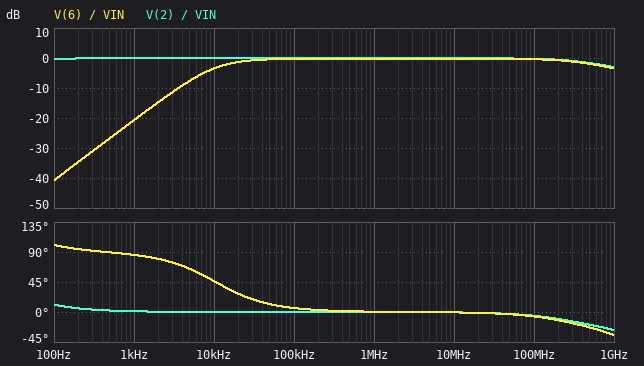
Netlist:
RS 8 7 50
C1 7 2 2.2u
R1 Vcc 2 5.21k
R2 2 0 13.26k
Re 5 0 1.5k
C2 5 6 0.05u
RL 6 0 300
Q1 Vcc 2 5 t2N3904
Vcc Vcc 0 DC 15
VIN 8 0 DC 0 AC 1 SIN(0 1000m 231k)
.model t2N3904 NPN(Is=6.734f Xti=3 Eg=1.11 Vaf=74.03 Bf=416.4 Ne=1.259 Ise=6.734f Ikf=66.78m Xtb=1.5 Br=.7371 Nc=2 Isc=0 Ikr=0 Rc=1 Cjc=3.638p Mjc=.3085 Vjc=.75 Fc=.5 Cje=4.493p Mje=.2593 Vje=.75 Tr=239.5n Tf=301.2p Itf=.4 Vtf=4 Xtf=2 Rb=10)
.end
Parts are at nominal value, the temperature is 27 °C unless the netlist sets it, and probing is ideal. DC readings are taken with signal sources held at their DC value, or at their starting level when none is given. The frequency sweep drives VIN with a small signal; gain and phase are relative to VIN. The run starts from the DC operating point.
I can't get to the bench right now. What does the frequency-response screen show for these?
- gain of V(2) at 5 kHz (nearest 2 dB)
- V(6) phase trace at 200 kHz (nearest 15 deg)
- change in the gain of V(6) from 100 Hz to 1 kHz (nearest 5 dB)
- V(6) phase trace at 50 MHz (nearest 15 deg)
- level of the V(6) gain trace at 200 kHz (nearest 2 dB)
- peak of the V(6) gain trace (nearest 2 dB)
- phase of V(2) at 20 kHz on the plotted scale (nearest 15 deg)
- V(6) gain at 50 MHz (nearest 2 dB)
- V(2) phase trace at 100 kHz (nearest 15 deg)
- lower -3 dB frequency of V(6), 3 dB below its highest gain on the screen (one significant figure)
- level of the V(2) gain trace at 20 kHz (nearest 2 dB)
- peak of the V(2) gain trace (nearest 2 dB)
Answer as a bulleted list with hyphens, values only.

- 0 dB
- 0 deg
- 20 dB
- 0 deg
- 0 dB
- 0 dB
- 0 deg
- 0 dB
- 0 deg
- 10 kHz
- 0 dB
- 0 dB
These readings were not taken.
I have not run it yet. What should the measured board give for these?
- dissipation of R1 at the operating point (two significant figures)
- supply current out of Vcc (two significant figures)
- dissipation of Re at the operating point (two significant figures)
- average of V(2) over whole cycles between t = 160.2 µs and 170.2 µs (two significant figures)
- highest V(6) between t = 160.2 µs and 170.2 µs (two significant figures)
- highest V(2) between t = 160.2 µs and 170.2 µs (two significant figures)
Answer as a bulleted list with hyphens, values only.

- 3.7 mW
- 7.4 mA
- 65 mW
- 11 V
- 970 mV
- 12 V
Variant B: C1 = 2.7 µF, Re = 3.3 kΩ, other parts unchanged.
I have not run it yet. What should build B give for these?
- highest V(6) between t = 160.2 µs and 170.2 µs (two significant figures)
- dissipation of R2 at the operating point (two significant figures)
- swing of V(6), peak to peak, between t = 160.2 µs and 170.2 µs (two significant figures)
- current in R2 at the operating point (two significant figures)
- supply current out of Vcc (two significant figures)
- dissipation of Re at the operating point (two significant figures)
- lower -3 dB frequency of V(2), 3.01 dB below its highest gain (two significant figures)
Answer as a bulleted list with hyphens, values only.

- 940 mV
- 8.6 mW
- 1.8 V
- 810 µA
- 3.8 mA
- 30 mW
- 16 Hz
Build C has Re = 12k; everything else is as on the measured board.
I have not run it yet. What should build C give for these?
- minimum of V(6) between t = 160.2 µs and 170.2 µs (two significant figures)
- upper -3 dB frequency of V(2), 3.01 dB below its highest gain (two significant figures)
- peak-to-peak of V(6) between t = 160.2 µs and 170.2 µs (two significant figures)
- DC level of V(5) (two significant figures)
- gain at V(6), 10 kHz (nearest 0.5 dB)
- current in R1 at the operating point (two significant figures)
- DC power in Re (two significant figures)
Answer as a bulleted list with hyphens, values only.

- -260 mV
- 1.1 GHz
- 850 mV
- 10 V
- -4.0 dB
- 820 µA
- 8.5 mW
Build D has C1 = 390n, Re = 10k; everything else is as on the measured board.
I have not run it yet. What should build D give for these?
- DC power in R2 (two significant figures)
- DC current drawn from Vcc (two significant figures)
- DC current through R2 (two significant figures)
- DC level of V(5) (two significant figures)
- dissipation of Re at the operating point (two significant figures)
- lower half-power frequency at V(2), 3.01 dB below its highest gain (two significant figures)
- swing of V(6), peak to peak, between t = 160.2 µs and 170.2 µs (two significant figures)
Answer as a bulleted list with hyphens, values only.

- 8.7 mW
- 1.8 mA
- 810 µA
- 10 V
- 10 mW
- 110 Hz
- 950 mV
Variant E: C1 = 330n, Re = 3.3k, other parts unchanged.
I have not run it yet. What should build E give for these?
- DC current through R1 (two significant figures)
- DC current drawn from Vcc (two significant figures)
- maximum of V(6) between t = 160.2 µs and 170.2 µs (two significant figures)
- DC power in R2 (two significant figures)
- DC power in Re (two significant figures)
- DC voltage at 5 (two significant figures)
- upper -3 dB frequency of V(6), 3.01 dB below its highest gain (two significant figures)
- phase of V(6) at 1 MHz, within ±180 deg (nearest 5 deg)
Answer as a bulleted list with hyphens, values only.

- 830 µA
- 3.8 mA
- 940 mV
- 8.6 mW
- 30 mW
- 10 V
- 1.0 GHz
- 0 deg
